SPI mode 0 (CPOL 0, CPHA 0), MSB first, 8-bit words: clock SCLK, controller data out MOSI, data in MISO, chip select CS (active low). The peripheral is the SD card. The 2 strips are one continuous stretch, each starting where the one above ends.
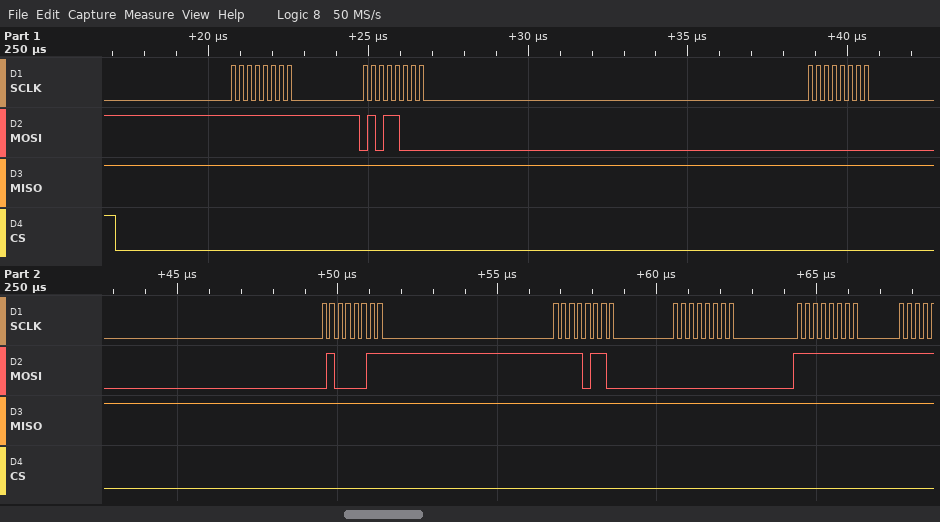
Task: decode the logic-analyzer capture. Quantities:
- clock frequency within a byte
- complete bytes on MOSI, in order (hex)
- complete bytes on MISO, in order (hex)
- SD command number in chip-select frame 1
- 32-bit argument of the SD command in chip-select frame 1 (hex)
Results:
4 MHz
FF 58 00 43 F6 00 FF
FF FF FF FF FF FF FF
CMD24
0x0043F600
